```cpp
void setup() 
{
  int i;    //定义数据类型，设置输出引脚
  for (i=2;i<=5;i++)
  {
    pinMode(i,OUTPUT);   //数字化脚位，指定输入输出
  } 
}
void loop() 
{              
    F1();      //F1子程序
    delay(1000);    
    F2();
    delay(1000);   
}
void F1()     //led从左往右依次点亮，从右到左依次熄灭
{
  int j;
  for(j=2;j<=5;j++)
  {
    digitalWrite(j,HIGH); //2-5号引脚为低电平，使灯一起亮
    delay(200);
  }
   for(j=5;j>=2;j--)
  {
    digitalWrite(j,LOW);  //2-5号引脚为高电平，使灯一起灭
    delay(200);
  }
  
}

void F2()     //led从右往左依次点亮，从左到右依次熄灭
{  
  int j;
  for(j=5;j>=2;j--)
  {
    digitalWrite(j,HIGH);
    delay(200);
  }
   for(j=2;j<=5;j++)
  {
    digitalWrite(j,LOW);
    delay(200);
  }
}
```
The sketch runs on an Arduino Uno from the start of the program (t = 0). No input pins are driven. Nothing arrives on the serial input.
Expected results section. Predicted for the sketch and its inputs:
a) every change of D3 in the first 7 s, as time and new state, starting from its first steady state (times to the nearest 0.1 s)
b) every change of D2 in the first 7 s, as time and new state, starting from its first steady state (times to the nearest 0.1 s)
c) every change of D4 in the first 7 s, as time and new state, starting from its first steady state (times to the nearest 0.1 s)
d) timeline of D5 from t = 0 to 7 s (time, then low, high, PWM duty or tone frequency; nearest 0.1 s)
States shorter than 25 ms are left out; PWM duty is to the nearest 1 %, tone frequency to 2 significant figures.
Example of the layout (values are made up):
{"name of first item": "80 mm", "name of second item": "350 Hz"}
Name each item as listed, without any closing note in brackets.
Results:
{"every change of D3 in the first 7 s, as time and new state, starting from its first steady state": "0 s low; 0.2 s high; 1.2 s low; 3 s high; 3.6 s low; 5.4 s high; 6.4 s low", "every change of D2 in the first 7 s, as time and new state, starting from its first steady state": "0 s high; 1.4 s low; 3.2 s high; 3.4 s low; 5.2 s high; 6.6 s low", "every change of D4 in the first 7 s, as time and new state, starting from its first steady state": "0 s low; 0.4 s high; 1 s low; 2.8 s high; 3.8 s low; 5.6 s high; 6.2 s low", "timeline of D5 from t = 0 to 7 s": "0 s low; 0.6 s high; 0.8 s low; 2.6 s high; 4 s low; 5.8 s high; 6 s low"}
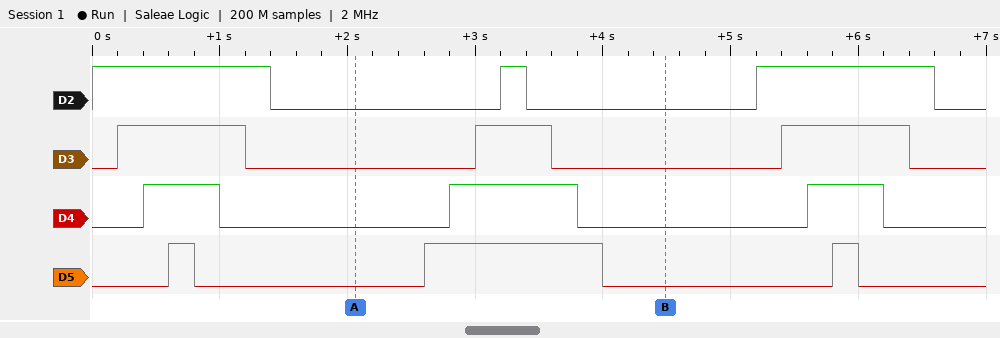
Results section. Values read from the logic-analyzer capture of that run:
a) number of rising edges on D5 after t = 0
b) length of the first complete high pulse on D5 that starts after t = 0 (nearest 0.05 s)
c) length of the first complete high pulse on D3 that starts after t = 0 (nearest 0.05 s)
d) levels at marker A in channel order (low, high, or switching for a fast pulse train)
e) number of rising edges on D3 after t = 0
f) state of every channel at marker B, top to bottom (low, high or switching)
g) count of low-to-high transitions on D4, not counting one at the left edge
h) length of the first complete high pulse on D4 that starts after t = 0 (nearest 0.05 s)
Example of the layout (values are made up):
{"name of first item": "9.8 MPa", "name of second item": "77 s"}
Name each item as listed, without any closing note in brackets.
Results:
{"number of rising edges on D5 after t = 0": "3", "length of the first complete high pulse on D5 that starts after t = 0": "0.20 s", "length of the first complete high pulse on D3 that starts after t = 0": "1.00 s", "levels at marker A in channel order": "D2 low, D3 low, D4 low, D5 low", "number of rising edges on D3 after t = 0": "3", "state of every channel at marker B, top to bottom": "D2 low, D3 low, D4 low, D5 low", "count of low-to-high transitions on D4, not counting one at the left edge": "3", "length of the first complete high pulse on D4 that starts after t = 0": "0.60 s"}
